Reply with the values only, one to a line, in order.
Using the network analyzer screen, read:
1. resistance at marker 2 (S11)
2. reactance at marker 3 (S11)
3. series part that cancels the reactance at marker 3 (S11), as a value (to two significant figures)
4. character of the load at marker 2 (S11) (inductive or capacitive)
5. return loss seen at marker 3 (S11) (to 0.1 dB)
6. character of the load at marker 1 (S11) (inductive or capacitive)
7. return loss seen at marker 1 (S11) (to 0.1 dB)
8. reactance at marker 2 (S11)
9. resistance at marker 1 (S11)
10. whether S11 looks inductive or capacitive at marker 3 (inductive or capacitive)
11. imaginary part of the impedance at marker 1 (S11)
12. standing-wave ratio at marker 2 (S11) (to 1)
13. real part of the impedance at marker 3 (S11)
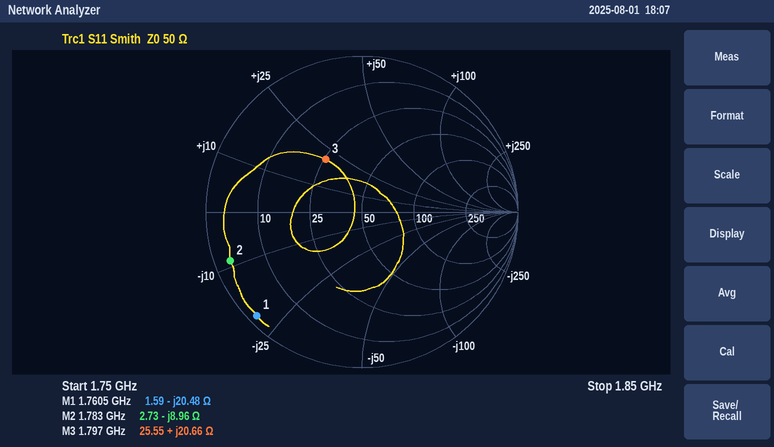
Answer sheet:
2.73 Ω
+20.66 Ω
4.3 pF
capacitive
7.8 dB
capacitive
0.5 dB
-8.96 Ω
1.59 Ω
inductive
-20.48 Ω
19
25.55 Ω
